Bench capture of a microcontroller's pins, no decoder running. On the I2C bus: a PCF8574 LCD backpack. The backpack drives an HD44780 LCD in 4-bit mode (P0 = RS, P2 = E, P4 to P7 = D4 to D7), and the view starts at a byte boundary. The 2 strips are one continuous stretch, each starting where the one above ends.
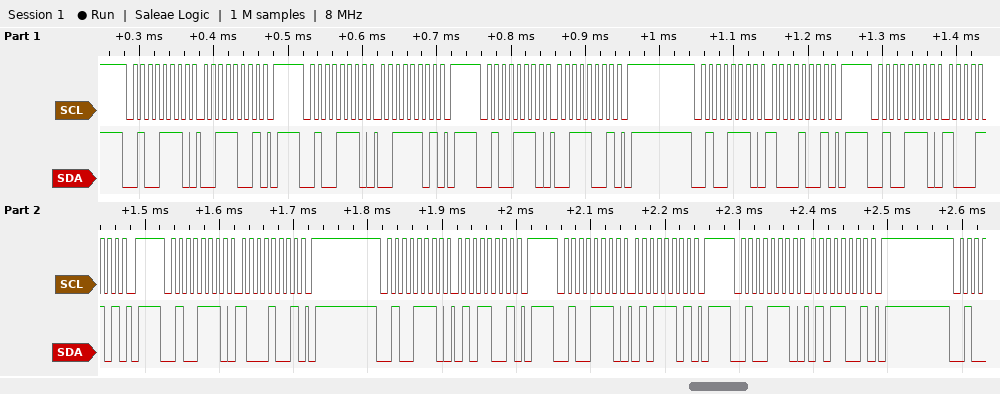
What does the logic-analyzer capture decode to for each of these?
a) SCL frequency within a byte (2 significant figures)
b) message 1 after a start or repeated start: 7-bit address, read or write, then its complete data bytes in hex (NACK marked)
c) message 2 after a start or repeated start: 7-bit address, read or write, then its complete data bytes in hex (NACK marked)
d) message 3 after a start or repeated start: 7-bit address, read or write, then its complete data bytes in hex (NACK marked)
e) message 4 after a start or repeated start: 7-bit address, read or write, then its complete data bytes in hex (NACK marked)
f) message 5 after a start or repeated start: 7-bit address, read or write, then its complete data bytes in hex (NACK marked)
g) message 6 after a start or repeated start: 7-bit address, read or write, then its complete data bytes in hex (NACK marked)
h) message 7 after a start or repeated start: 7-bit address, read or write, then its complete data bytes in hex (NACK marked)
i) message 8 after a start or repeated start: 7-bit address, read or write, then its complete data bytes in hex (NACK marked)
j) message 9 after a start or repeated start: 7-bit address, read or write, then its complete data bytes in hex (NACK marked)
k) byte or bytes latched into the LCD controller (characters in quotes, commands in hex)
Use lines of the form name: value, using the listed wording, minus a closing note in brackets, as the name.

SCL frequency within a byte: 100 kHz
message 1 after a start or repeated start: 7-bit address, read or write, then its complete data bytes in hex: 0x27 write: 39
message 2 after a start or repeated start: 7-bit address, read or write, then its complete data bytes in hex: 0x27 write: 3D
message 3 after a start or repeated start: 7-bit address, read or write, then its complete data bytes in hex: 0x27 write: 39
message 4 after a start or repeated start: 7-bit address, read or write, then its complete data bytes in hex: 0x27 write: 89
message 5 after a start or repeated start: 7-bit address, read or write, then its complete data bytes in hex: 0x27 write: 8D
message 6 after a start or repeated start: 7-bit address, read or write, then its complete data bytes in hex: 0x27 write: 89
message 7 after a start or repeated start: 7-bit address, read or write, then its complete data bytes in hex: 0x27 write: 59
message 8 after a start or repeated start: 7-bit address, read or write, then its complete data bytes in hex: 0x27 write: 5D
message 9 after a start or repeated start: 7-bit address, read or write, then its complete data bytes in hex: 0x27 write: 59
byte or bytes latched into the LCD controller: '8'
